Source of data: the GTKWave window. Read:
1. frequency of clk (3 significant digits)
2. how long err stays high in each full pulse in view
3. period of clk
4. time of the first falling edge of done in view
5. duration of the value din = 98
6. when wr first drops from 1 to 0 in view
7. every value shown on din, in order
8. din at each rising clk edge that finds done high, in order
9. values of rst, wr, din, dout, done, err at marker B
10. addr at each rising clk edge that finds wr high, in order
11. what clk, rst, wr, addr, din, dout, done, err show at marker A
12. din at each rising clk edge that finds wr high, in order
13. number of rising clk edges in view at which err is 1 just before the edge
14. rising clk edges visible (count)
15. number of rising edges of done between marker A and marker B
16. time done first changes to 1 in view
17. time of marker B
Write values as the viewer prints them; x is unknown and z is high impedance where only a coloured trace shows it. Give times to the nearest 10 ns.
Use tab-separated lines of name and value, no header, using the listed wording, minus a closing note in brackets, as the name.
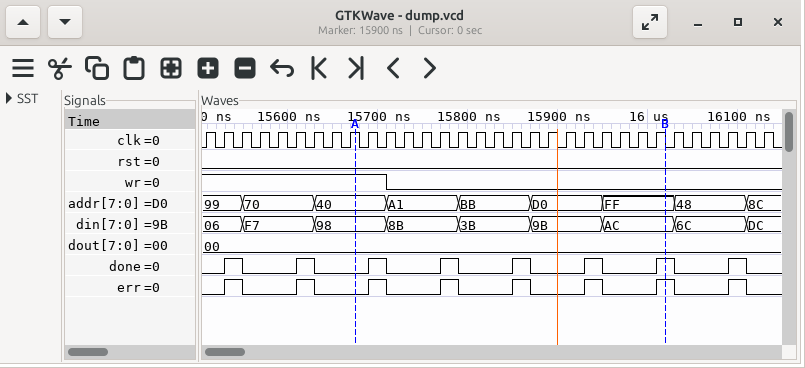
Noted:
frequency of clk	50.0 MHz
how long err stays high in each full pulse in view	20 ns, 20 ns, 20 ns, 20 ns, 20 ns, 20 ns, 20 ns, 20 ns
period of clk	20 ns
time of the first falling edge of done in view	15550 ns
duration of the value din = 98	80 ns
when wr first drops from 1 to 0 in view	15710 ns
every value shown on din, in order	06, F7, 98, 8B, 3B, 9B, AC, 6C, DC
din at each rising clk edge that finds done high, in order	06, F7, 98, 8B, 3B, 9B, AC, 6C
values of rst, wr, din, dout, done, err at marker B	rst=0, wr=0, din=AC, dout=00, done=1, err=1
addr at each rising clk edge that finds wr high, in order	99, 99, 99, 70, 70, 70, 70, 40, 40, 40, 40
what clk, rst, wr, addr, din, dout, done, err show at marker A	clk=1, rst=0, wr=1, addr=40, din=98, dout=00, done=0, err=0
din at each rising clk edge that finds wr high, in order	06, 06, 06, F7, F7, F7, F7, 98, 98, 98, 98
number of rising clk edges in view at which err is 1 just before the edge	8
rising clk edges visible	32
number of rising edges of done between marker A and marker B	5
time done first changes to 1 in view	15530 ns
time of marker B	16020 ns
